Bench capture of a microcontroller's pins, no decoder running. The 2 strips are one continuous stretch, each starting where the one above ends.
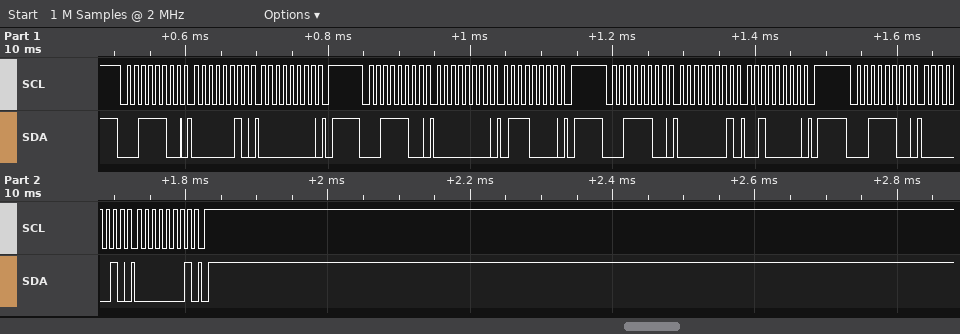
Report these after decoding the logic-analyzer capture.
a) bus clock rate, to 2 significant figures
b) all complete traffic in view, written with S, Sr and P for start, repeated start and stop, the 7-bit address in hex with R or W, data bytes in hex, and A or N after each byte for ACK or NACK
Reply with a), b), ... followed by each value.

a) 100 kHz
b) S 1EW A 02 A 00 A P S 1EW A 00 A 70 A P S 1EW A 01 A 20 A P S 1EW A 02 A 01 A P
